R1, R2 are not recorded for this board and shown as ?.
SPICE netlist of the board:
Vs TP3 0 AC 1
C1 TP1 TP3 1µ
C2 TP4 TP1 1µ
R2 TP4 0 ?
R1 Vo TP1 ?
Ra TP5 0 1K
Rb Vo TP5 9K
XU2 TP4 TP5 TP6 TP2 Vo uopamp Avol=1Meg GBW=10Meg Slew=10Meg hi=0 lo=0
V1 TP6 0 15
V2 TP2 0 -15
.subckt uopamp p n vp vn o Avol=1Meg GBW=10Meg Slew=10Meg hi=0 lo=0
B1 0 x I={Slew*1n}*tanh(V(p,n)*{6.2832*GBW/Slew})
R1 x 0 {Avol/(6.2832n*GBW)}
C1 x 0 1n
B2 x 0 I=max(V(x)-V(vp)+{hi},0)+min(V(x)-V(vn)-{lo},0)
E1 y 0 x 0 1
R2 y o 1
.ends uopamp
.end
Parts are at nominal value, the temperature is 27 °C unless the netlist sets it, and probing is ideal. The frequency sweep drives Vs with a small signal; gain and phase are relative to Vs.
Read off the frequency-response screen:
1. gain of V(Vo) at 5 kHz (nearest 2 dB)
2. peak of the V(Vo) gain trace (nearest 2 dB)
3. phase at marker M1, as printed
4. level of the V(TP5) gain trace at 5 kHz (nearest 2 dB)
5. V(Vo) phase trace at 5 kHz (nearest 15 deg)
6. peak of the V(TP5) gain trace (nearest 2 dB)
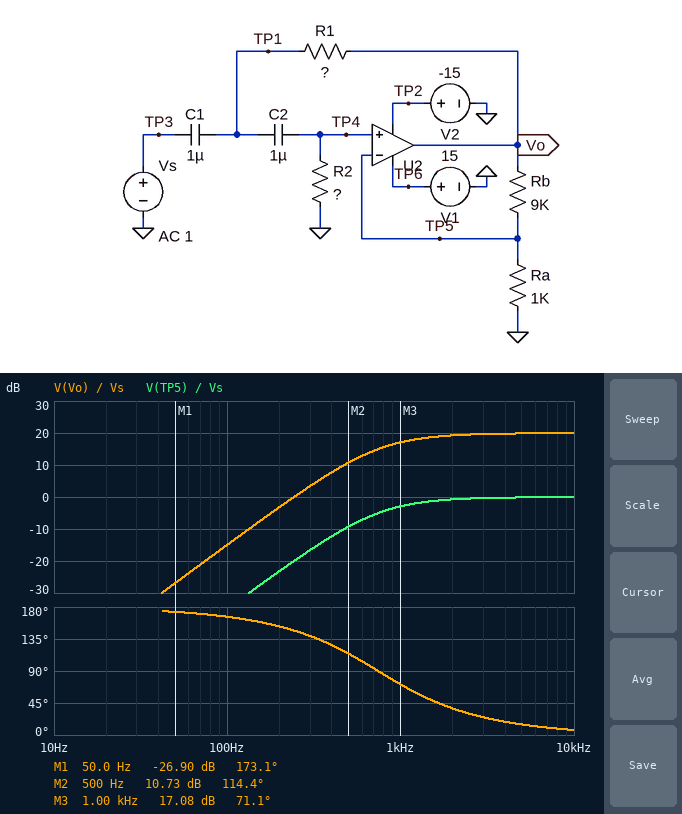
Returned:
20 dB
20 dB
173.1 deg
0 dB
15 deg
0 dB
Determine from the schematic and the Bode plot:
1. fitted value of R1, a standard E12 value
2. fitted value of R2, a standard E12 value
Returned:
560 Ω
82 Ω
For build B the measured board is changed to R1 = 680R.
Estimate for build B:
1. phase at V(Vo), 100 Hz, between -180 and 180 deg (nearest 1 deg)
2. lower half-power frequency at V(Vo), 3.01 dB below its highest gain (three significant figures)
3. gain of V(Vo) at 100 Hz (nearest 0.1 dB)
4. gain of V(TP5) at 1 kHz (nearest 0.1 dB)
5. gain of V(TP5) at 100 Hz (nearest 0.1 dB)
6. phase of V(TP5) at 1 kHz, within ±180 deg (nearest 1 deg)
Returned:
158 deg
1.52 kHz
-13.6 dB
-5.4 dB
-33.6 dB
73 deg
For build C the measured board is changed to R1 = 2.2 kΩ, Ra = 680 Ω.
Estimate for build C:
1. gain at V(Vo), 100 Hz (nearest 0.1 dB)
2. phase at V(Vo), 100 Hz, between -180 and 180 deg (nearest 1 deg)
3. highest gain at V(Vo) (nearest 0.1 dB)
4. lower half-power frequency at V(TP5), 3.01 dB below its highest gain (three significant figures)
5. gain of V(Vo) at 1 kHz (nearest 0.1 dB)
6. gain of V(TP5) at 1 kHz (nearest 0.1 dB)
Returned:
-7.0 dB
114 deg
23.0 dB
2.85 kHz
13.4 dB
-9.7 dB
